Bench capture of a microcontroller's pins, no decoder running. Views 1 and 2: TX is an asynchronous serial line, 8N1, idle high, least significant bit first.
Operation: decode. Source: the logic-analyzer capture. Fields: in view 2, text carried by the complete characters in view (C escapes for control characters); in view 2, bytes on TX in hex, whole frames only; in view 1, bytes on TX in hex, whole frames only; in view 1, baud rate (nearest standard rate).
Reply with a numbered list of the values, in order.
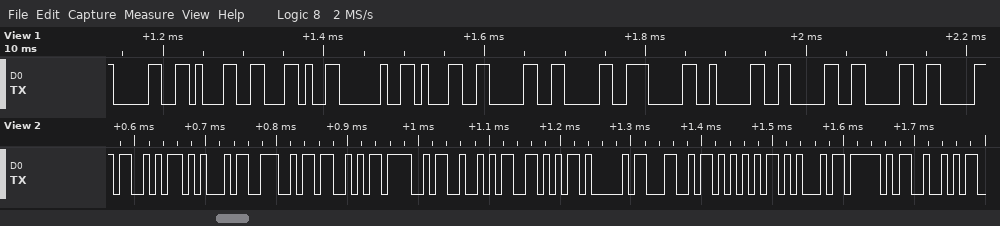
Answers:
1. "SENSORVALUE_R"
2. 53 45 4E 53 4F 52 56 41 4C 55 45 5F 52
3. 30 31 2C 20 31 30 30 30 30 30 30
4. 115200 baud
